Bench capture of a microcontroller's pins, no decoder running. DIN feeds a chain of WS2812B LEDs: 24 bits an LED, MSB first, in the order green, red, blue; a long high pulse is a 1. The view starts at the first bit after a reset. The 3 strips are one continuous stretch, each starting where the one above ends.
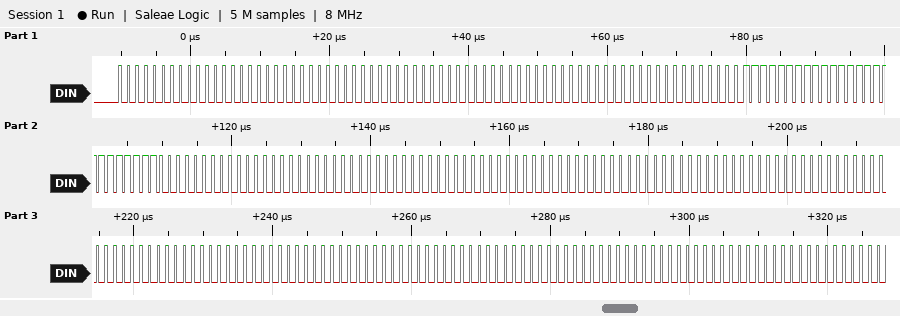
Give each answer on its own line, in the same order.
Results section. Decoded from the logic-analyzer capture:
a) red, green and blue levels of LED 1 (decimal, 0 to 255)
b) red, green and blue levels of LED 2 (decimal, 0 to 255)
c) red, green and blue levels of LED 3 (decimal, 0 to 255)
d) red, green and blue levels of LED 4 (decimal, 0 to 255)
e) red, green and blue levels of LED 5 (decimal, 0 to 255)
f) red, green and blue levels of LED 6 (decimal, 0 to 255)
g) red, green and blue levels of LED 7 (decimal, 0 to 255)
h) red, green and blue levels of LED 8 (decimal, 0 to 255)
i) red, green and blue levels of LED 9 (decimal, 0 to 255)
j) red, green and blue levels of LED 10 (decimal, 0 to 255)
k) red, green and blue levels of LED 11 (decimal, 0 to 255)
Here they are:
0, 0, 0
0, 0, 0
0, 0, 0
255, 255, 255
0, 0, 0
0, 0, 0
0, 0, 0
0, 0, 0
0, 0, 0
0, 0, 0
0, 0, 0
